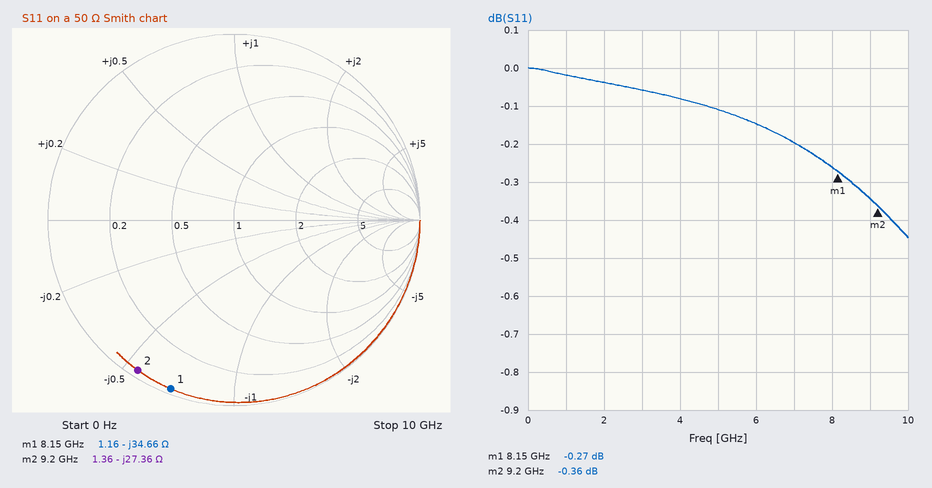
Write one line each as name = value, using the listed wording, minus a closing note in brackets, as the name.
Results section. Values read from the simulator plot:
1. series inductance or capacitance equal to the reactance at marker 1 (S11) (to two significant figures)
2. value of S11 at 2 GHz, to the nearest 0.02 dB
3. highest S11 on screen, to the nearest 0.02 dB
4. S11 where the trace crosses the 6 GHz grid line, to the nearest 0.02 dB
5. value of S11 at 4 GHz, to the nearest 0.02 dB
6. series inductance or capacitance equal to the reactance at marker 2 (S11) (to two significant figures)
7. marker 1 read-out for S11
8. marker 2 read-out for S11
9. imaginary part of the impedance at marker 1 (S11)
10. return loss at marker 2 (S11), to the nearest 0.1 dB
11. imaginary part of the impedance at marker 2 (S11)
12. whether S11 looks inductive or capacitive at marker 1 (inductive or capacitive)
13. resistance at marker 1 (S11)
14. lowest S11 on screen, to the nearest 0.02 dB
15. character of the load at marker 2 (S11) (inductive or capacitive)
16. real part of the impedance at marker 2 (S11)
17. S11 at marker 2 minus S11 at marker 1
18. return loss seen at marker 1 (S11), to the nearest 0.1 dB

series inductance or capacitance equal to the reactance at marker 1 (S11) = 560 fF
value of S11 at 2 GHz, to the nearest 0.02 dB = -0.04 dB
highest S11 on screen, to the nearest 0.02 dB = 0.00 dB
S11 where the trace crosses the 6 GHz grid line, to the nearest 0.02 dB = -0.14 dB
value of S11 at 4 GHz, to the nearest 0.02 dB = -0.08 dB
series inductance or capacitance equal to the reactance at marker 2 (S11) = 630 fF
marker 1 read-out for S11 = -0.27 dB
marker 2 read-out for S11 = -0.36 dB
imaginary part of the impedance at marker 1 = -34.66 Ω
return loss at marker 2 (S11), to the nearest 0.1 dB = 0.4 dB
imaginary part of the impedance at marker 2 = -27.36 Ω
whether S11 looks inductive or capacitive at marker 1 = capacitive
resistance at marker 1 = 1.16 Ω
lowest S11 on screen, to the nearest 0.02 dB = -0.44 dB
character of the load at marker 2 (S11) = capacitive
real part of the impedance at marker 2 = 1.36 Ω
S11 at marker 2 minus S11 at marker 1 = -0.09 dB
return loss seen at marker 1 (S11), to the nearest 0.1 dB = 0.3 dB
